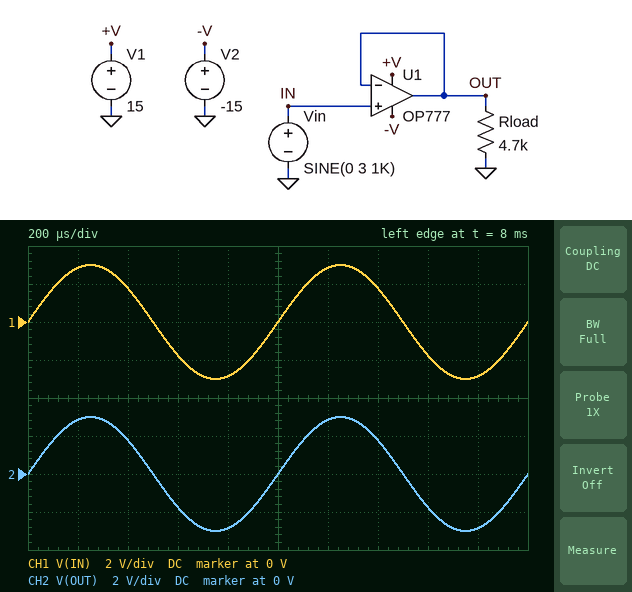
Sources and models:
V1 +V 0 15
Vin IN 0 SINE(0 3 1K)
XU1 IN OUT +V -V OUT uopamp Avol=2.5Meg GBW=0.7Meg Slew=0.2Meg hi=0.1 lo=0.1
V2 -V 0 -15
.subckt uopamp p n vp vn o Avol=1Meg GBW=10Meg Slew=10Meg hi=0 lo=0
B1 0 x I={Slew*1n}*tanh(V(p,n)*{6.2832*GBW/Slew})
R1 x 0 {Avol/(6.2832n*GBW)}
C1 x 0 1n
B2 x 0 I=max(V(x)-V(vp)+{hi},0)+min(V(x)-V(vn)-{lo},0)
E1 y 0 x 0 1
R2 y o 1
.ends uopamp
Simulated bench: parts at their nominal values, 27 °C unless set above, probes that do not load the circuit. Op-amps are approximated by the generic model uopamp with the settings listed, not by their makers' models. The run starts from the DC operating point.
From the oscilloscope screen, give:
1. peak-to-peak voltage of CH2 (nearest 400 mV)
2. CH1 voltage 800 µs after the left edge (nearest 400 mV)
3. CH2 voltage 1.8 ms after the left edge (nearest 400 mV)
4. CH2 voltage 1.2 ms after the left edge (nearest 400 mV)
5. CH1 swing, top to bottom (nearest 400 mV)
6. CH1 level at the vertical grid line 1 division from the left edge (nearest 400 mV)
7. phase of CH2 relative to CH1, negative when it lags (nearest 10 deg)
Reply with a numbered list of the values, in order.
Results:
1. 6.0 V
2. -2.8 V
3. -2.8 V
4. 2.8 V
5. 6.0 V
6. 2.8 V
7. 0 deg
